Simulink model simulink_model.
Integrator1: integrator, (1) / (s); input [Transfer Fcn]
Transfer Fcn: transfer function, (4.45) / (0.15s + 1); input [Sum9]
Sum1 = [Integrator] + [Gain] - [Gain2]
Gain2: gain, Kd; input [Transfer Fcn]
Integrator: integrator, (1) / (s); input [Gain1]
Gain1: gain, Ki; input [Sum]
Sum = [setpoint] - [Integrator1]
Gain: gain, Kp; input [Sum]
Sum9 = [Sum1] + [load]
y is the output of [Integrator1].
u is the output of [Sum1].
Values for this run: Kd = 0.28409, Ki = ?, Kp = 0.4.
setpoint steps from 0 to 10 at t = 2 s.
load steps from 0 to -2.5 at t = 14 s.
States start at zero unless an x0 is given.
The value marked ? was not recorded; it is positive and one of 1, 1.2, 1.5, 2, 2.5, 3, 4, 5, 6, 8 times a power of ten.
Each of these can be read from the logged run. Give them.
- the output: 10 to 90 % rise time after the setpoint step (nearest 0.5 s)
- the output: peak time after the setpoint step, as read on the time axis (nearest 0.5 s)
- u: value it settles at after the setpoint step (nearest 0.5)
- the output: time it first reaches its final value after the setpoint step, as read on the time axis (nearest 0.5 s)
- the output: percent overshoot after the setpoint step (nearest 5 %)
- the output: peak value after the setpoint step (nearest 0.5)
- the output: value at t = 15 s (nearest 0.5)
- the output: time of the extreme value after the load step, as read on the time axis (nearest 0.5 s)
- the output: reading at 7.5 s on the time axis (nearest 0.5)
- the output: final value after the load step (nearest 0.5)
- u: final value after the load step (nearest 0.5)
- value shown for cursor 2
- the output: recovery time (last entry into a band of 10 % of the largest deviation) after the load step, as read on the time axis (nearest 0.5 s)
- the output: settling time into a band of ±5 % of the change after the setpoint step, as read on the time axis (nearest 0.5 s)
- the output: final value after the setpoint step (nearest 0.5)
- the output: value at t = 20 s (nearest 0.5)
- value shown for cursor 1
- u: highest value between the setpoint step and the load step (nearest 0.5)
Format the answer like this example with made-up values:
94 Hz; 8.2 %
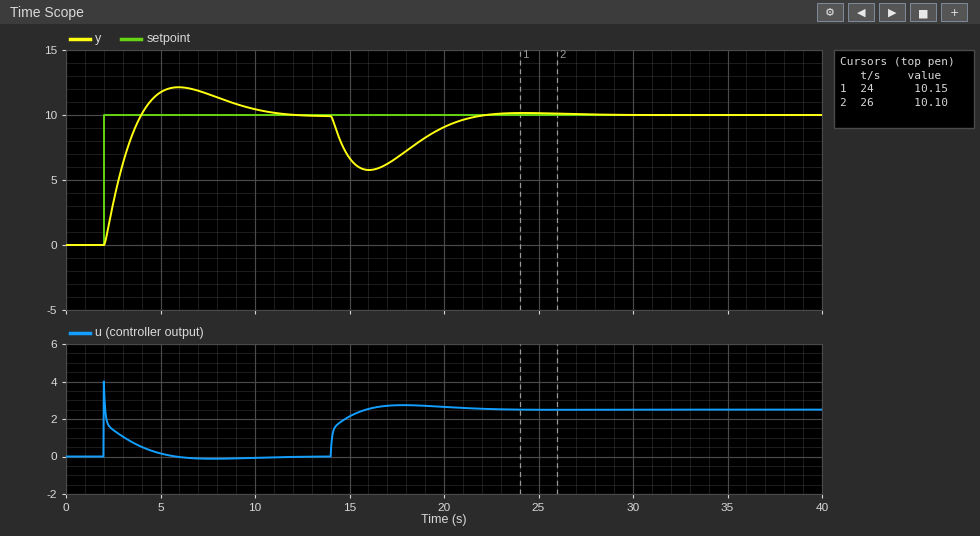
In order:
1.5 s; 6.0 s; 0.0; 4.0 s; 20 %; 12.0; 6.5; 16.0 s; 11.5; 10.0; 2.5; 10.10; 21.0 s; 10.0 s; 10.0; 9.0; 10.15; 4.0
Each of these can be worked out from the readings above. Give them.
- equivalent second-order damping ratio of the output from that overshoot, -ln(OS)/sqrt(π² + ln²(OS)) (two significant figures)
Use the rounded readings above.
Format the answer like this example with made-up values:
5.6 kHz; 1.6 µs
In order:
0.46
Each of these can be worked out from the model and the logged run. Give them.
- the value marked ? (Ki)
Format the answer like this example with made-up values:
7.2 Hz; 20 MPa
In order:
0.15
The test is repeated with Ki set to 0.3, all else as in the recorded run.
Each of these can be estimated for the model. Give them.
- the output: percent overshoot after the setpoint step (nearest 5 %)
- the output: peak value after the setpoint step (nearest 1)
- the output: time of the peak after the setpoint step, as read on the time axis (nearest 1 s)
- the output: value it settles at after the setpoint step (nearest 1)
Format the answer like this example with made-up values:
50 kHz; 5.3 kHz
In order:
30 %; 13; 5 s; 10
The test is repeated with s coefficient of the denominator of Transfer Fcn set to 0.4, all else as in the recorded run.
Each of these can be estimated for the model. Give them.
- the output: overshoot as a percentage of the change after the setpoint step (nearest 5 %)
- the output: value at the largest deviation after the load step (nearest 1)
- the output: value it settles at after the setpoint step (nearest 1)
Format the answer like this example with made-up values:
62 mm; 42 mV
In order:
25 %; 6; 10
